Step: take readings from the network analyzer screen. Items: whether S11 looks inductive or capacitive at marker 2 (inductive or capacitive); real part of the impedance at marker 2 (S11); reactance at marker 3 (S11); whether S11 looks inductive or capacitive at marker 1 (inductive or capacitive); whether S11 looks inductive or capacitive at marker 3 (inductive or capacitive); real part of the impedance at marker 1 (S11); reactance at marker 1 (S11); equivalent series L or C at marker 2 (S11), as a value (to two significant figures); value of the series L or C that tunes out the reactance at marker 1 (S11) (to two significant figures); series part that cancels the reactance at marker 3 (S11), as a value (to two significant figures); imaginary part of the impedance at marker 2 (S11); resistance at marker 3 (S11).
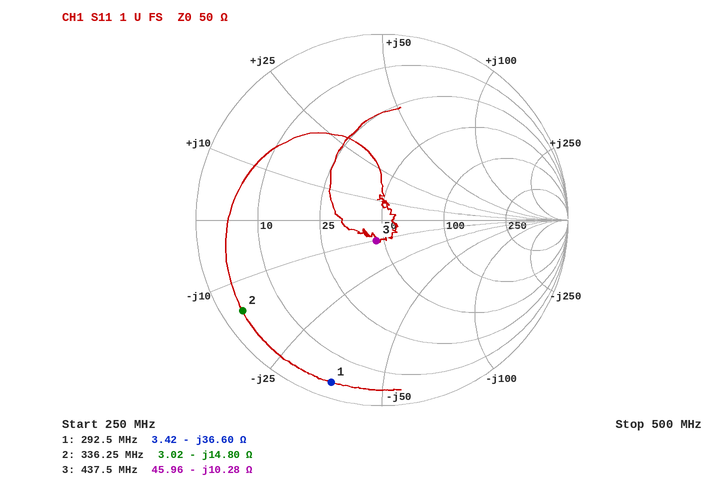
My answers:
capacitive
3.02 Ω
-10.28 Ω
capacitive
capacitive
3.42 Ω
-36.60 Ω
32 pF
20 nH
3.7 nH
-14.80 Ω
45.96 Ω
